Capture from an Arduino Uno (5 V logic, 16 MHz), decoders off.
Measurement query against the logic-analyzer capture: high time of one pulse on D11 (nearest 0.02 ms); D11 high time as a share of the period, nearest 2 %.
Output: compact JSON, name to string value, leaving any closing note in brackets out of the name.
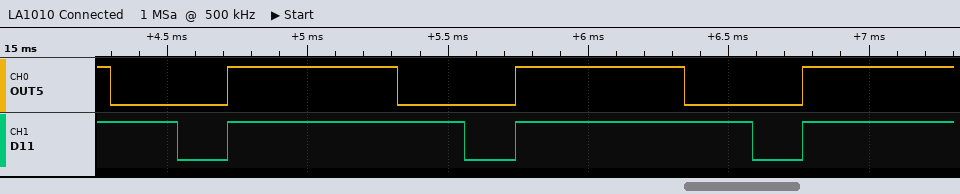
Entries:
{"high time of one pulse on D11": "0.84 ms", "D11 high time as a share of the period, nearest 2 %": "82 %"}
